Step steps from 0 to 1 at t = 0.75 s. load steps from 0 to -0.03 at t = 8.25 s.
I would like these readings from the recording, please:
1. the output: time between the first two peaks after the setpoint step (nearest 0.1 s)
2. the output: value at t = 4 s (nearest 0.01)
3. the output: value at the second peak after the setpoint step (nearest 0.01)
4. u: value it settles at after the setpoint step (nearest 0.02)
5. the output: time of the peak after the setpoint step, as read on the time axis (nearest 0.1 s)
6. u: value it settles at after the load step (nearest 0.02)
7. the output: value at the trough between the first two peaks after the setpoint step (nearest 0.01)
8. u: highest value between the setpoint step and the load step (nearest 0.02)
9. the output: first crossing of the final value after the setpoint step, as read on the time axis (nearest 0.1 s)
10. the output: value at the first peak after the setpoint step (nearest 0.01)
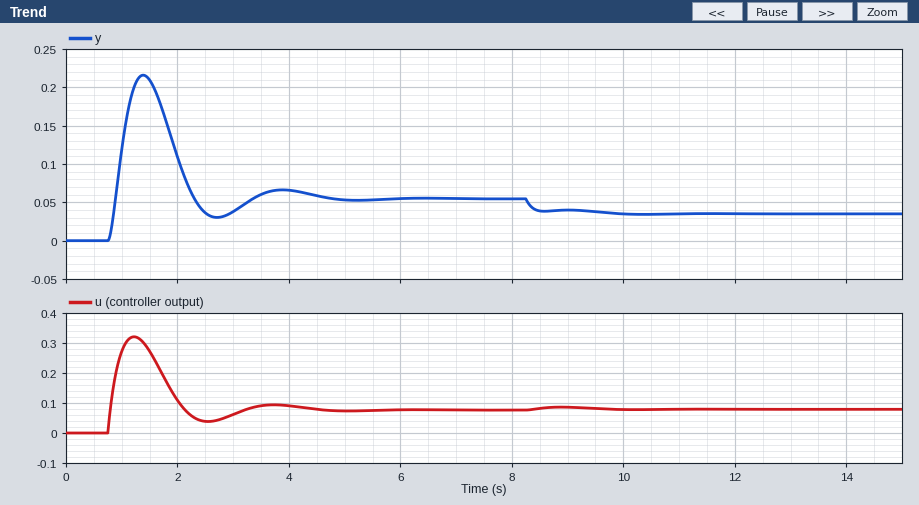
2.5 s
0.07
0.07
0.08
1.4 s
0.08
0.03
0.32
0.9 s
0.22
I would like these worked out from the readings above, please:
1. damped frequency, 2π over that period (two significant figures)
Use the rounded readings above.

2.5 rad/s
